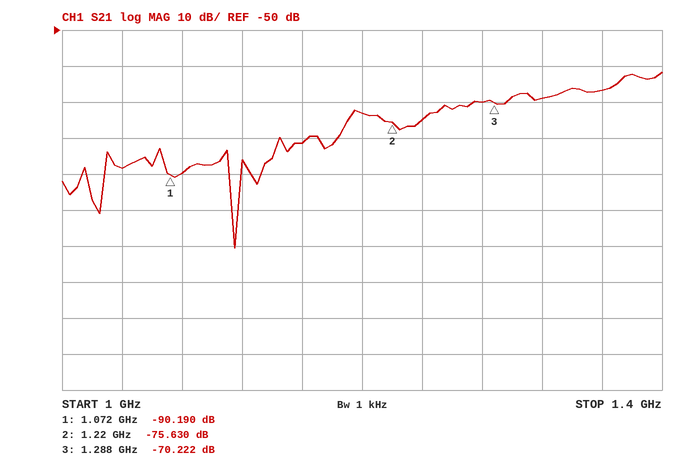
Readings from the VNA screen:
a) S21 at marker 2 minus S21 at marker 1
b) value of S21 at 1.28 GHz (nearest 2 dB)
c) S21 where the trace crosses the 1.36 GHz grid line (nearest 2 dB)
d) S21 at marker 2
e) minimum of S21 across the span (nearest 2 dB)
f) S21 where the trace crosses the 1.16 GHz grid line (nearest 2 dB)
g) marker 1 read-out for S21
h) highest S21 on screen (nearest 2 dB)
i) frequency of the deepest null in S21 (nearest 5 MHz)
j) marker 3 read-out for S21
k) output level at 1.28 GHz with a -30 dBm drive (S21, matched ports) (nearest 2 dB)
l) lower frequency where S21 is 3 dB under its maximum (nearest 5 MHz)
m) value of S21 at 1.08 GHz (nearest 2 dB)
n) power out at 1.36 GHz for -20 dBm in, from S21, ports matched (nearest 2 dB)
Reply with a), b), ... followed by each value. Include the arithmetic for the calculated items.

a) -75.63 − (-90.19) = 14.560 dB
b) -70 dB
c) -66 dB
d) -75.630 dB
e) -110 dB
f) -82 dB
g) -90.190 dB
h) -62 dB
i) 1.115 GHz
j) -70.222 dB
k) -30 dBm + (-70 dB) = -100 dBm
l) 1.370 GHz
m) -90 dB
n) -20 dBm + (-66 dB) = -86 dBm
